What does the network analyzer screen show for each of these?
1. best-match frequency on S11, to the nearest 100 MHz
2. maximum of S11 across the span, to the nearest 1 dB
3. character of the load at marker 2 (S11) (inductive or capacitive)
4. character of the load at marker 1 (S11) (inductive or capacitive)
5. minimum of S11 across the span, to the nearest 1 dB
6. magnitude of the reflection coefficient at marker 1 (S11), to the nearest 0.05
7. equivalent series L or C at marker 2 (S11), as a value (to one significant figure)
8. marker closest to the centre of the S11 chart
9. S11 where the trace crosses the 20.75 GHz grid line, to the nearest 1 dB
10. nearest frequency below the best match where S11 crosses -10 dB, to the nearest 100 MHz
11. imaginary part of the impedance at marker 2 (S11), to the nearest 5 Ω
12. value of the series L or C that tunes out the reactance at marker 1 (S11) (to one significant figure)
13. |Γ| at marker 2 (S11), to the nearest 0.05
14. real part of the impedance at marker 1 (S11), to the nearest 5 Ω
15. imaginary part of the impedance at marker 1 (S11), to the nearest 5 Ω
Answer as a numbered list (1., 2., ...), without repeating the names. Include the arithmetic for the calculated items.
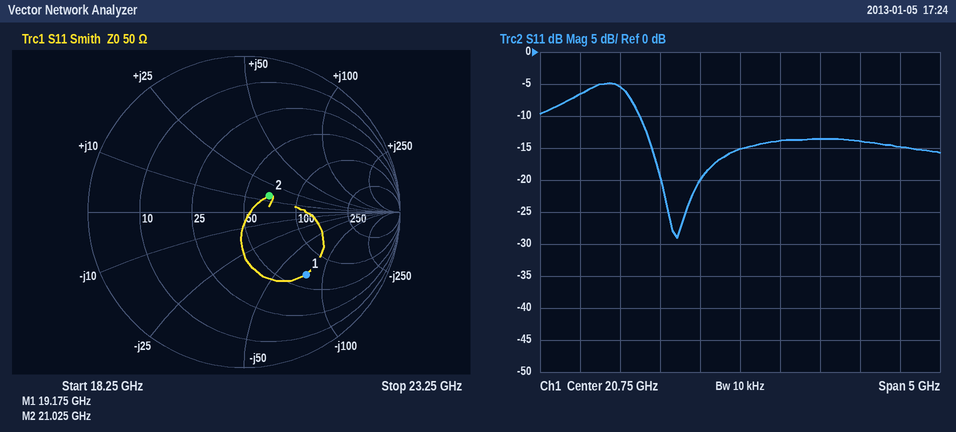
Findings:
1. 20.0 GHz
2. -5 dB
3. inductive
4. capacitive
5. -29 dB
6. 0.55
7. L = 15 Ω/(2π × 21.025 GHz) ≈ 114 pH, so 100 pH to one significant figure
8. marker 2
9. -15 dB
10. 19.5 GHz
11. +15 Ω
12. L = 75 Ω/(2π × 19.175 GHz) ≈ 623 pH, so 600 pH to one significant figure
13. 0.20
14. 65 Ω
15. -75 Ω
